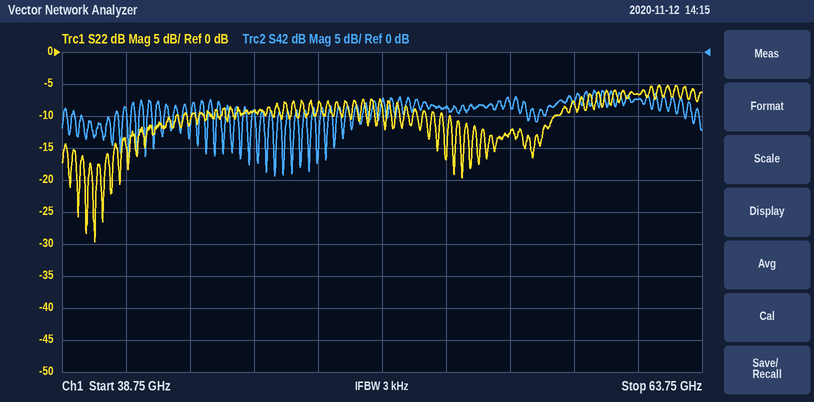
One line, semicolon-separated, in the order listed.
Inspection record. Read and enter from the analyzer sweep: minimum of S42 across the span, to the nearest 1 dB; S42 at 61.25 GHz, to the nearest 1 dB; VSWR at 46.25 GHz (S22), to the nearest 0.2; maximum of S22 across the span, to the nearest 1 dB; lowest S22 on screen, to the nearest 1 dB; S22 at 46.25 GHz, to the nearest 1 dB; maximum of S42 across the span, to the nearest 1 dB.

-19 dB; -7 dB; 2.0; -5 dB; -30 dB; -9 dB; -6 dB
